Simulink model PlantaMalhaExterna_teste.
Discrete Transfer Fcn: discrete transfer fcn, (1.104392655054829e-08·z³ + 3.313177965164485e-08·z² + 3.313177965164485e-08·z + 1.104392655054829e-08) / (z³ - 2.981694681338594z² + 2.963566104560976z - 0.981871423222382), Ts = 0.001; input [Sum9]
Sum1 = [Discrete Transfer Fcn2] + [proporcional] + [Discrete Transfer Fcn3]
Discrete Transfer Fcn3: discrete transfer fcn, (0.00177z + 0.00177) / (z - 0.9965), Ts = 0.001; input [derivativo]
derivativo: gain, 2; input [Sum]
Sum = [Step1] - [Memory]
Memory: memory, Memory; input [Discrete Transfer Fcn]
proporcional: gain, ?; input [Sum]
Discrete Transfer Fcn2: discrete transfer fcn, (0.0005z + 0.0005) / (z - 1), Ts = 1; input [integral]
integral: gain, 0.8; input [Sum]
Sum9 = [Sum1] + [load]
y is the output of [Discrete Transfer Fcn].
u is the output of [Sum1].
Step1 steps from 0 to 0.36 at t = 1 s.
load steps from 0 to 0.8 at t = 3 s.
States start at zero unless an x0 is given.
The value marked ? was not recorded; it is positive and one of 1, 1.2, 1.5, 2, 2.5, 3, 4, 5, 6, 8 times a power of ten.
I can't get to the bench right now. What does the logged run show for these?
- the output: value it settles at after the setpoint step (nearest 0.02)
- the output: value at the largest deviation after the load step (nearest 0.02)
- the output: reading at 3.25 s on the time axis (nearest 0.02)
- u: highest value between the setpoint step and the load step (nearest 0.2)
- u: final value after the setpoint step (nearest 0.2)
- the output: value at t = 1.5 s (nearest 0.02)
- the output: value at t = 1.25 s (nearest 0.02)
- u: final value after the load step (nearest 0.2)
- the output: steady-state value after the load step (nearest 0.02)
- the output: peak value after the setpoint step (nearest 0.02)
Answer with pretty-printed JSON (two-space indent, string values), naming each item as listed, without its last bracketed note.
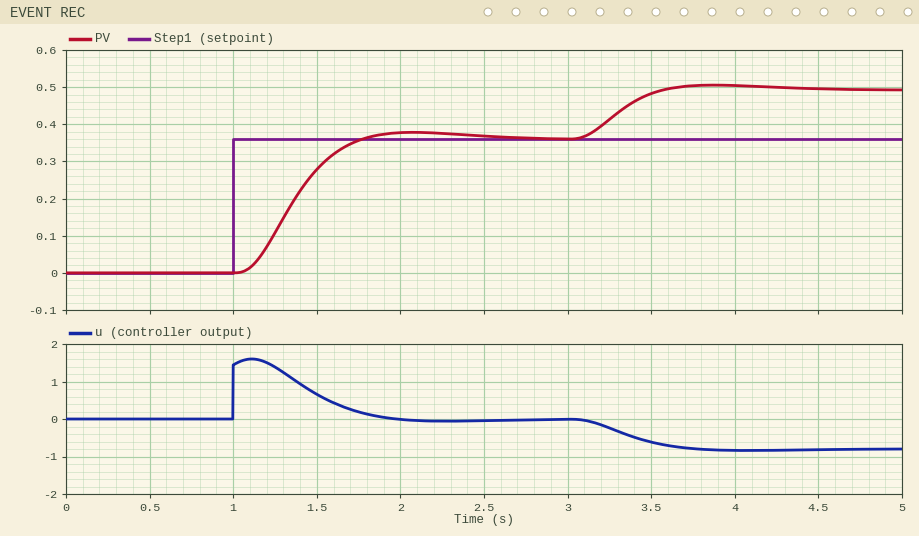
{
  "the output: value it settles at after the setpoint step": "0.36",
  "the output: value at the largest deviation after the load step": "0.50",
  "the output: reading at 3.25 s on the time axis": "0.42",
  "u: highest value between the setpoint step and the load step": "1.6",
  "u: final value after the setpoint step": "0.0",
  "the output: value at t = 1.5 s": "0.28",
  "the output: value at t = 1.25 s": "0.10",
  "u: final value after the load step": "-0.8",
  "the output: steady-state value after the load step": "0.50",
  "the output: peak value after the setpoint step": "0.38"
}
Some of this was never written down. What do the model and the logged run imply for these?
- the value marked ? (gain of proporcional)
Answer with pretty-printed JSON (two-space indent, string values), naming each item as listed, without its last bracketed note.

{
  "the value marked ?": "4"
}
